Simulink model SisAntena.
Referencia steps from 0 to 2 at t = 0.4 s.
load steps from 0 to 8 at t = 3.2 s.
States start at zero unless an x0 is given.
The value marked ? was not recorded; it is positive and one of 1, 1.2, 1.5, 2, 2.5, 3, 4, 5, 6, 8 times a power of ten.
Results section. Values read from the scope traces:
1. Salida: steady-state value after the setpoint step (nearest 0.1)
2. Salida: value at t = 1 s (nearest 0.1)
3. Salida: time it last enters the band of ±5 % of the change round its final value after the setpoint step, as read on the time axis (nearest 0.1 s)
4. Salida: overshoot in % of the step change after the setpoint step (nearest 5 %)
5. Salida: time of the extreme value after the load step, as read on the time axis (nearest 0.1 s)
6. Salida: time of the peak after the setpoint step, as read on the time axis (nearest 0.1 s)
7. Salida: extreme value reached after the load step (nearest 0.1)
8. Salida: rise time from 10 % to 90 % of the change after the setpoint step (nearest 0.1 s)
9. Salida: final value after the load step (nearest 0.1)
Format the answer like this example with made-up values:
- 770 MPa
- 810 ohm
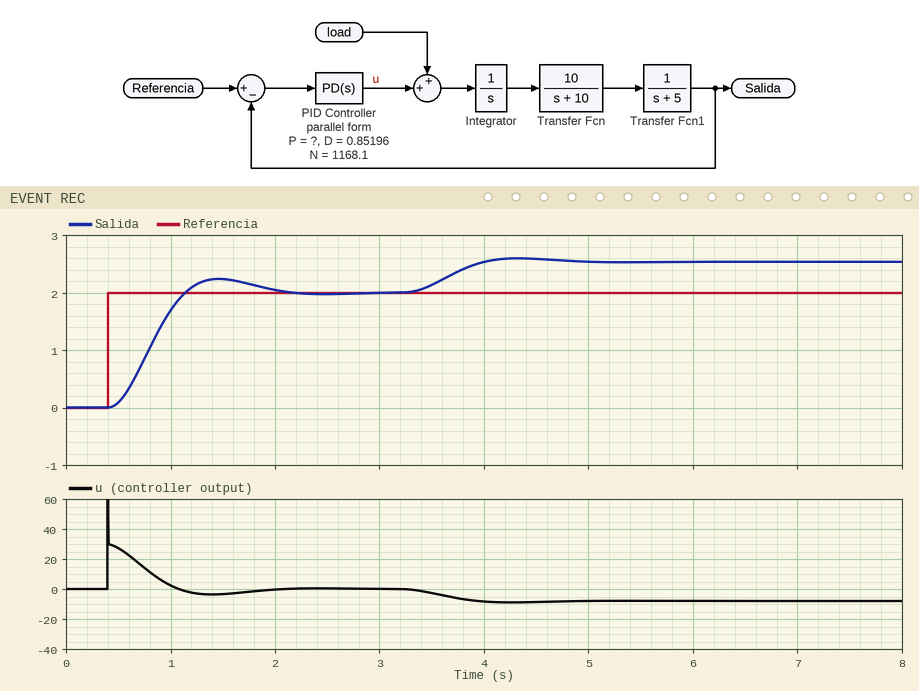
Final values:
- 2.0
- 1.7
- 1.9 s
- 10 %
- 4.3 s
- 1.5 s
- 2.6
- 0.5 s
- 2.5
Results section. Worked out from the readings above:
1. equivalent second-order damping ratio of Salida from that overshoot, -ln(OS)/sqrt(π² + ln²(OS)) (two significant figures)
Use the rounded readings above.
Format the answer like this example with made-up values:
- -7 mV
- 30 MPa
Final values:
- 0.59
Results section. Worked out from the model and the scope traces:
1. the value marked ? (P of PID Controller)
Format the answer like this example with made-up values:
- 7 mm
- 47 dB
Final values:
- 15
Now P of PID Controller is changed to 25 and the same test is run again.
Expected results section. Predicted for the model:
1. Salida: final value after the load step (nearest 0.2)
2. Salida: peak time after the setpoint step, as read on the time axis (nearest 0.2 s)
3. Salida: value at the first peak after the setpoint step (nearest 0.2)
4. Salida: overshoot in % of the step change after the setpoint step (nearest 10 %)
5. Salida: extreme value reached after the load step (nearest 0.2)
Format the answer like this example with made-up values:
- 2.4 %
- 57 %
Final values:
- 2.4
- 1.2 s
- 2.6
- 30 %
- 2.4
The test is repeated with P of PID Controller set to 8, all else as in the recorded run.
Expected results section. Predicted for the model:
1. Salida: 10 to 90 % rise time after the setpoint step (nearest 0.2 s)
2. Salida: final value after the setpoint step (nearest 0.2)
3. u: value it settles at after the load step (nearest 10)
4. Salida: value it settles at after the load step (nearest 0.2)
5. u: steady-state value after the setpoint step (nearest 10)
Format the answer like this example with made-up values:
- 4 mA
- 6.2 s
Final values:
- 1.0 s
- 2.0
- -10
- 3.0
- 0
